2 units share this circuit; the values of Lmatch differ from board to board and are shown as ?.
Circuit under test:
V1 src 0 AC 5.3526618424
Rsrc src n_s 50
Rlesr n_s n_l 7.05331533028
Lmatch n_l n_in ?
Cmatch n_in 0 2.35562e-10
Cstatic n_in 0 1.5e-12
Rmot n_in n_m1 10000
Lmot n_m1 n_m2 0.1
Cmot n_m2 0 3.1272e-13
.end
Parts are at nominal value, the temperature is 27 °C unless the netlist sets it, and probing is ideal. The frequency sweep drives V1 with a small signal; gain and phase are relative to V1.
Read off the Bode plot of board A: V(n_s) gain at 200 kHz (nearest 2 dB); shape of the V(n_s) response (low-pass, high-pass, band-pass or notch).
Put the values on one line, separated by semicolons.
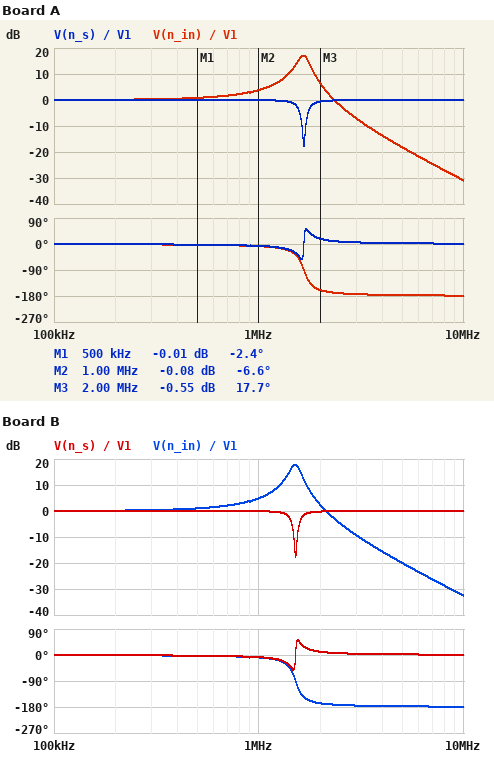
0 dB; notch
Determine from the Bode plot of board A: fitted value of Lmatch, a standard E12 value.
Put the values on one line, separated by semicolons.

39 µH
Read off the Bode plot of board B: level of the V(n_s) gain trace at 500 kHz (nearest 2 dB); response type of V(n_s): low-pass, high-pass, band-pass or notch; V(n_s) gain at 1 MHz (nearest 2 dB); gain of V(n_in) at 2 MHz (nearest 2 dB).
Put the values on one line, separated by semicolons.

0 dB; notch; 0 dB; 2 dB
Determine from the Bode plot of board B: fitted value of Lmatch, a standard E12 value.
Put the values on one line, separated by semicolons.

47 µH
